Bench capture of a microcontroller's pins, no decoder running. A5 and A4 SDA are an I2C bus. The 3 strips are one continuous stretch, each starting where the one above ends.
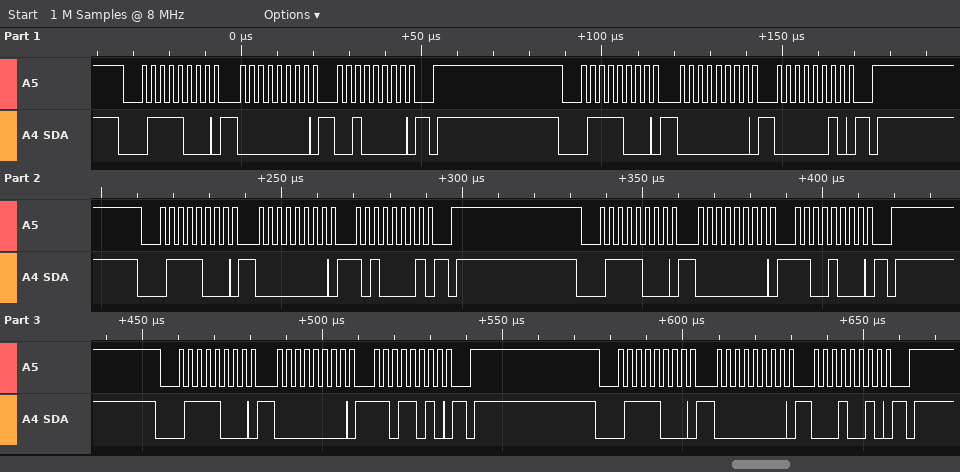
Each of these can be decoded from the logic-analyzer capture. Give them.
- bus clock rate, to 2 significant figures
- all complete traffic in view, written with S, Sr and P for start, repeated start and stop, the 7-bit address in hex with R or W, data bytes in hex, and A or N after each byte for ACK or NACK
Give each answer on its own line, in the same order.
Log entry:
400 kHz
S 3CW A 00 A 20 A P S 3CW A 00 A 02 A P S 3CW A 00 A A1 A P S 3CW A 00 A C8 A P S 3CW A 00 A DA A P S 3CW A 00 A 12 A P
